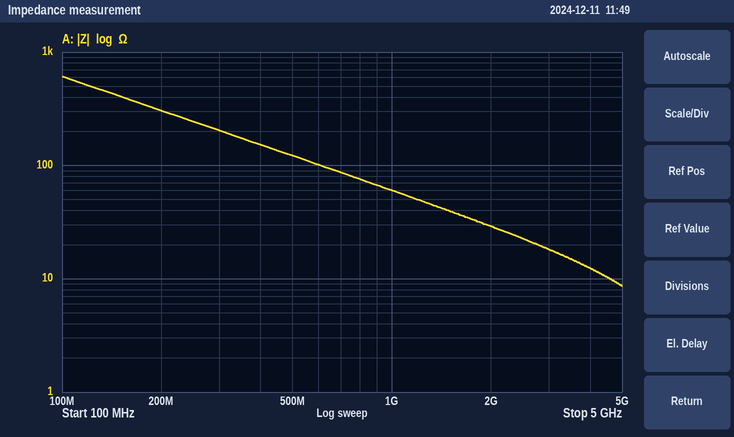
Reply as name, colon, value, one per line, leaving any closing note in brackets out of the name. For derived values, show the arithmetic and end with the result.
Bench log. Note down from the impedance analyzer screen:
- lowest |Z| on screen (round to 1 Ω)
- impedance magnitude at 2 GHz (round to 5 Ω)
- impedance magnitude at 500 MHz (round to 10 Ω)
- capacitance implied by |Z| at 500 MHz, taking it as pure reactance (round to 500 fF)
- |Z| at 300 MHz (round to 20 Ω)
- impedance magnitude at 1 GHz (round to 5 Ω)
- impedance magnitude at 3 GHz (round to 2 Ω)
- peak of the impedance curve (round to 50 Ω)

lowest |Z| on screen: 9 Ω
impedance magnitude at 2 GHz: 30 Ω
impedance magnitude at 500 MHz: 120 Ω
capacitance implied by |Z| at 500 MHz, taking it as pure reactance: C = 1/(2π × 500 MHz × 120 Ω) ≈ 2.65 pF, so 2.5 pF to the nearest 500 fF
|Z| at 300 MHz: 200 Ω
impedance magnitude at 1 GHz: 60 Ω
impedance magnitude at 3 GHz: 18 Ω
peak of the impedance curve: 600 Ω
